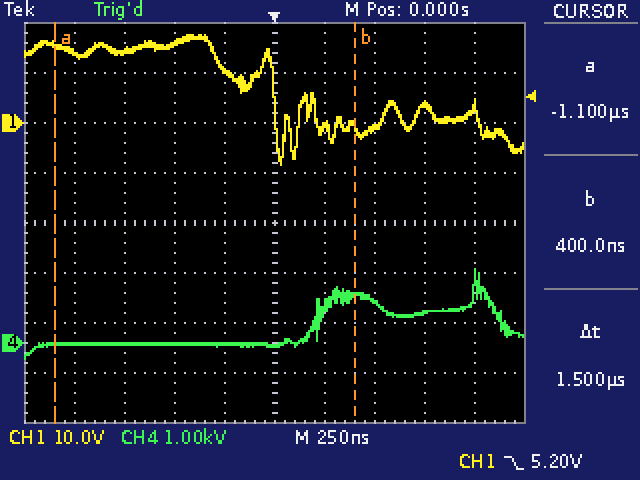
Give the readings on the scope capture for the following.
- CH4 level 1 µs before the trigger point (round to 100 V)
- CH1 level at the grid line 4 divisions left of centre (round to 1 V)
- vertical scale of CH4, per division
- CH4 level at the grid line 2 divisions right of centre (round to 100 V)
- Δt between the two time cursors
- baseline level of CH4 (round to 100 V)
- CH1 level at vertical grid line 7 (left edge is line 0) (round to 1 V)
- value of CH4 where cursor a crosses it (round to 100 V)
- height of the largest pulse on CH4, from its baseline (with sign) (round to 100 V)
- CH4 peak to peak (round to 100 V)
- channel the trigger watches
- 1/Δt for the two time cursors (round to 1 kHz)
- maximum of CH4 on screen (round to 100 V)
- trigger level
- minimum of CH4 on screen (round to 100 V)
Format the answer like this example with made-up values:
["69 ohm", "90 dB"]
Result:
["0.0 kV", "14 V", "1 kV", "800 V", "1.5 µs", "0.0 kV", "-1 V", "0.0 kV", "+1.5 kV", "1.8 kV", "CH1", "667 kHz", "1.5 kV", "5.20 V", "-300 V"]
